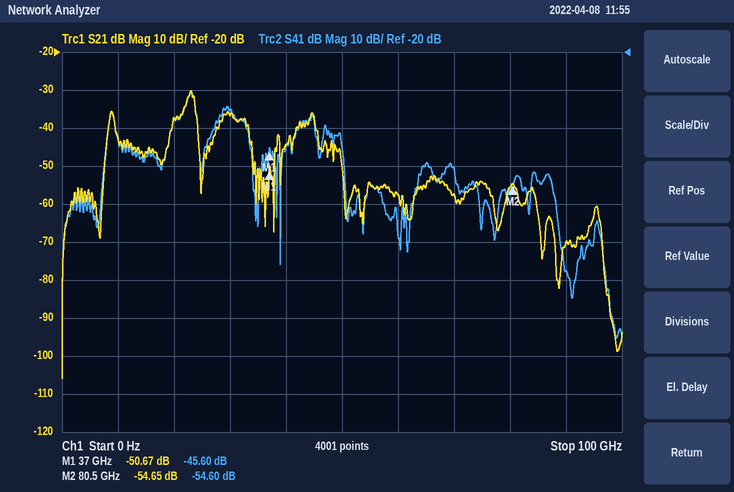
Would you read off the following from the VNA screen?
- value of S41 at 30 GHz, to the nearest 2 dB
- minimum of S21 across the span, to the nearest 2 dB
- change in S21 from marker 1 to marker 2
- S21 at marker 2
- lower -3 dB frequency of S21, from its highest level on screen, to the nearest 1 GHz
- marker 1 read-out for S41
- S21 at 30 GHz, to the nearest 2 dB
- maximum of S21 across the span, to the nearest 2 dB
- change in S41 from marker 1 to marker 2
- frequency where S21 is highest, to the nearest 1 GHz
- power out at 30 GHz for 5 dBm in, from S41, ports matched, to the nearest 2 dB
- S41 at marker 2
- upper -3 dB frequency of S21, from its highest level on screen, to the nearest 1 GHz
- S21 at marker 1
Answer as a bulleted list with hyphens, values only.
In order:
- -36 dB
- -106 dB
- -3.98 dB
- -54.65 dB
- 22 GHz
- -45.60 dB
- -36 dB
- -30 dB
- -9.00 dB
- 23 GHz
- -30 dBm
- -54.60 dB
- 24 GHz
- -50.67 dB
